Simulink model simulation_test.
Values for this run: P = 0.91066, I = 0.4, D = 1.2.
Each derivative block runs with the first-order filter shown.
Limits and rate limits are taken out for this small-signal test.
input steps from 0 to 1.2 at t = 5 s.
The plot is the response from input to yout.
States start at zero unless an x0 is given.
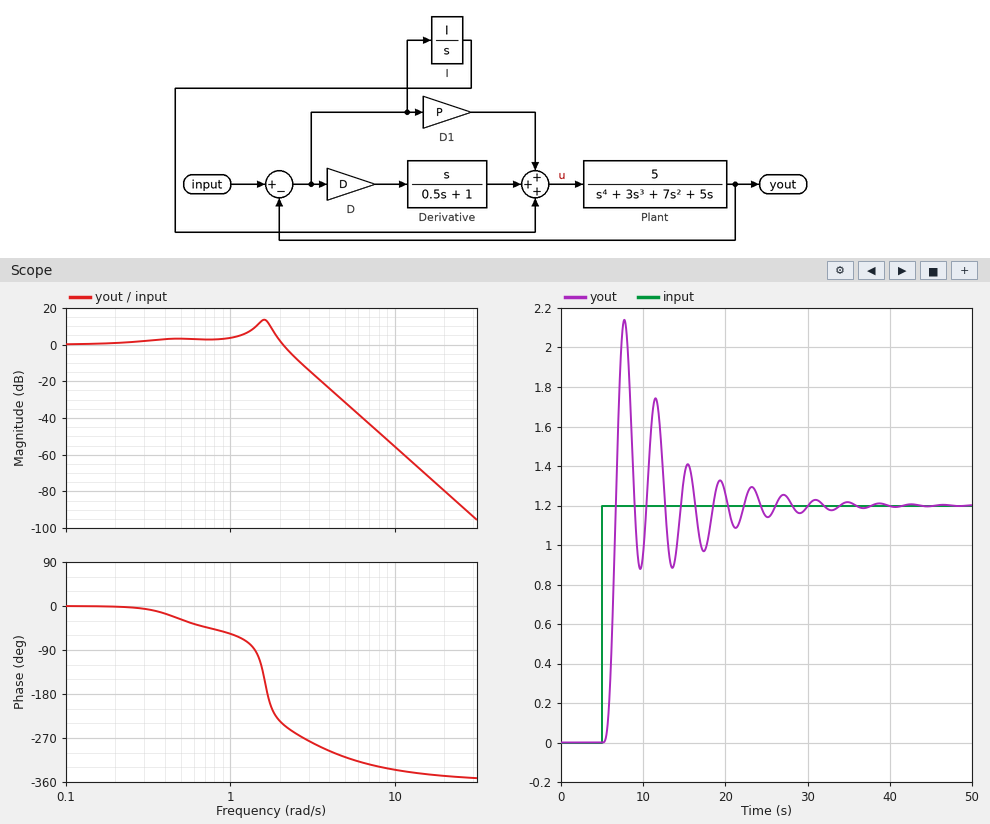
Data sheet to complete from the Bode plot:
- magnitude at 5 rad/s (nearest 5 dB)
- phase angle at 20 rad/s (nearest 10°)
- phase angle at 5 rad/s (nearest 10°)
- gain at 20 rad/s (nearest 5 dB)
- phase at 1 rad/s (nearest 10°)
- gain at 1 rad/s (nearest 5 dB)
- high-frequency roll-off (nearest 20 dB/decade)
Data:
-30 dB
-350°
-310°
-80 dB
-60°
5 dB
-80 dB/decade
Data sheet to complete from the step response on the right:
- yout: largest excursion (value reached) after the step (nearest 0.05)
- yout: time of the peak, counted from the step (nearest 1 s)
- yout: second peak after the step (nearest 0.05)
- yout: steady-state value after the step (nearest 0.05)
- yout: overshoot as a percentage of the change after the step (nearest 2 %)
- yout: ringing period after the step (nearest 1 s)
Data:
2.15
3 s
1.75
1.20
78 %
4 s
